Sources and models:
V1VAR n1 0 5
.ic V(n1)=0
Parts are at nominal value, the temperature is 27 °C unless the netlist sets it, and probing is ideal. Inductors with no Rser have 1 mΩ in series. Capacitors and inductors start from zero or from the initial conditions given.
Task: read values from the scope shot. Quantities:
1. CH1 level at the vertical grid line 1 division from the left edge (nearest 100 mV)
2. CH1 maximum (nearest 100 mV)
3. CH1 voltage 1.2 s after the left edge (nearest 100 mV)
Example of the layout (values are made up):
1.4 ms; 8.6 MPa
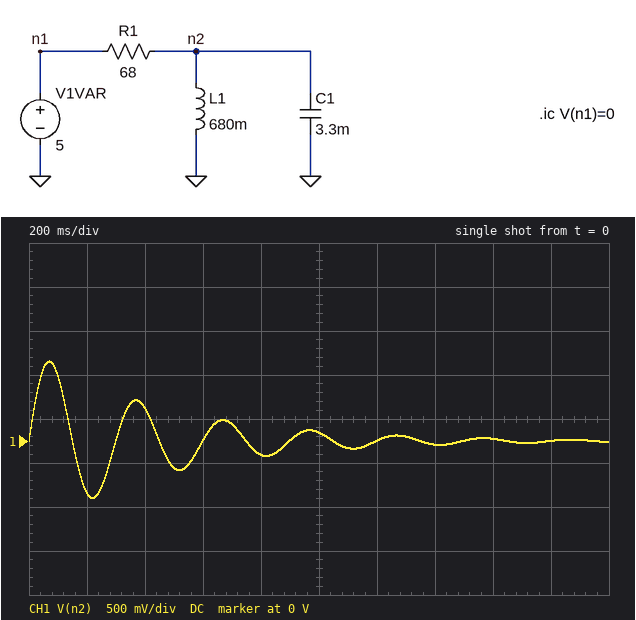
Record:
-600 mV; 900 mV; 0 V
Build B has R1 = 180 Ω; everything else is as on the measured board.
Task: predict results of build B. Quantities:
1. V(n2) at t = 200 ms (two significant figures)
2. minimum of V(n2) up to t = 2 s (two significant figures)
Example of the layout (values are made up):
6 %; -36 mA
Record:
-300 mV; -330 mV
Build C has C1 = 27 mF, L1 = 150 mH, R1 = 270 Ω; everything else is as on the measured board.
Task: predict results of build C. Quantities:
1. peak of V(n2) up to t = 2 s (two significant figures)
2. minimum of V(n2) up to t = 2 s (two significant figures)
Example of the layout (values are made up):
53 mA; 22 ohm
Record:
43 mV; -43 mV
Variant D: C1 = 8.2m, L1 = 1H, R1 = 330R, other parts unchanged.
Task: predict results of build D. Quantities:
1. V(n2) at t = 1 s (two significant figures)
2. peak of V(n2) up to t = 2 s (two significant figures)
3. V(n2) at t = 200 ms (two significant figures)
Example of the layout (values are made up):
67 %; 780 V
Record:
-140 mV; 160 mV; 130 mV
